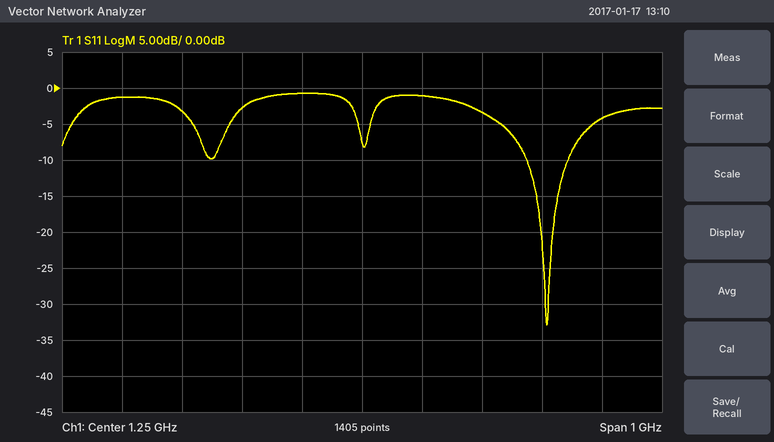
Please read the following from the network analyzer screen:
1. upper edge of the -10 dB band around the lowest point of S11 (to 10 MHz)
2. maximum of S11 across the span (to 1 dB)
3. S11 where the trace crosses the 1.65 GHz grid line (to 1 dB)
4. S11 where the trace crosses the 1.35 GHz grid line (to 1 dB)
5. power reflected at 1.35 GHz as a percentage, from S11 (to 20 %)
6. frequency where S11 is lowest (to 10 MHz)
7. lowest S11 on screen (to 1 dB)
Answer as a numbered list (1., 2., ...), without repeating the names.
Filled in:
1. 1.59 GHz
2. -1 dB
3. -4 dB
4. -1 dB
5. 80 %
6. 1.56 GHz
7. -33 dB
